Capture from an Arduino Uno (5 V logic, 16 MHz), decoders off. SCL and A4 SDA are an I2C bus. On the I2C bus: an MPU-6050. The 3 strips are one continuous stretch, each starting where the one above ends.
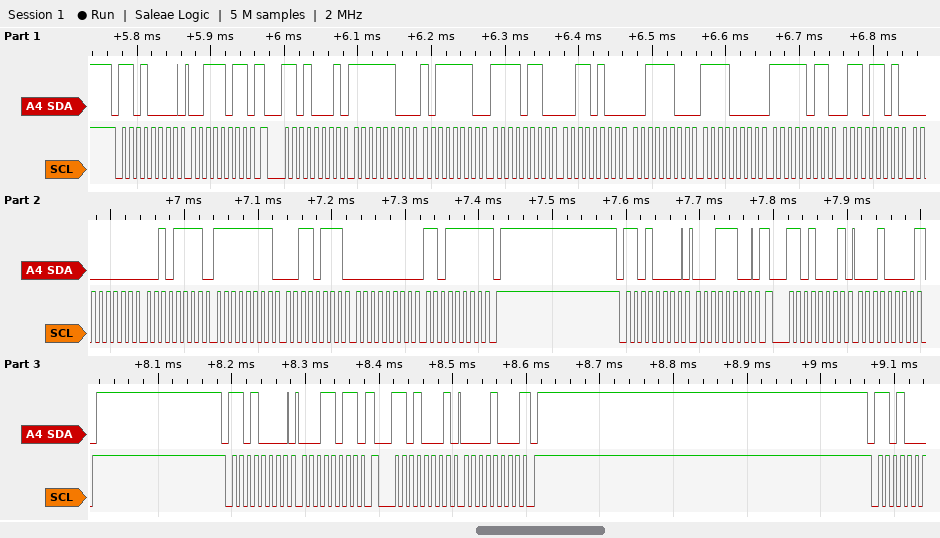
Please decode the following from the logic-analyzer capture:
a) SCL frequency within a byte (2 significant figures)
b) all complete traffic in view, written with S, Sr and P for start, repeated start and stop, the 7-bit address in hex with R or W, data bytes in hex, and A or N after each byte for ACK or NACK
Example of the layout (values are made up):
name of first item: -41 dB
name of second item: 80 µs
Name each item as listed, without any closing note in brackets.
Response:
SCL frequency within a byte: 100 kHz
all complete traffic in view, written with S, Sr and P for start, repeated start and stop, the 7-bit address in hex with R or W, data bytes in hex, and A or N after each byte for ACK or NACK: S 68W A 3B A Sr 68R A FC A BE A F6 A 34 A 3C A F0 A FB A 6D A 00 A 2F A FF A 37 A 00 A DF N P S 68W A 1C A Sr 68R A 10 N P S 68W A 1B A Sr 68R A 08 N P
